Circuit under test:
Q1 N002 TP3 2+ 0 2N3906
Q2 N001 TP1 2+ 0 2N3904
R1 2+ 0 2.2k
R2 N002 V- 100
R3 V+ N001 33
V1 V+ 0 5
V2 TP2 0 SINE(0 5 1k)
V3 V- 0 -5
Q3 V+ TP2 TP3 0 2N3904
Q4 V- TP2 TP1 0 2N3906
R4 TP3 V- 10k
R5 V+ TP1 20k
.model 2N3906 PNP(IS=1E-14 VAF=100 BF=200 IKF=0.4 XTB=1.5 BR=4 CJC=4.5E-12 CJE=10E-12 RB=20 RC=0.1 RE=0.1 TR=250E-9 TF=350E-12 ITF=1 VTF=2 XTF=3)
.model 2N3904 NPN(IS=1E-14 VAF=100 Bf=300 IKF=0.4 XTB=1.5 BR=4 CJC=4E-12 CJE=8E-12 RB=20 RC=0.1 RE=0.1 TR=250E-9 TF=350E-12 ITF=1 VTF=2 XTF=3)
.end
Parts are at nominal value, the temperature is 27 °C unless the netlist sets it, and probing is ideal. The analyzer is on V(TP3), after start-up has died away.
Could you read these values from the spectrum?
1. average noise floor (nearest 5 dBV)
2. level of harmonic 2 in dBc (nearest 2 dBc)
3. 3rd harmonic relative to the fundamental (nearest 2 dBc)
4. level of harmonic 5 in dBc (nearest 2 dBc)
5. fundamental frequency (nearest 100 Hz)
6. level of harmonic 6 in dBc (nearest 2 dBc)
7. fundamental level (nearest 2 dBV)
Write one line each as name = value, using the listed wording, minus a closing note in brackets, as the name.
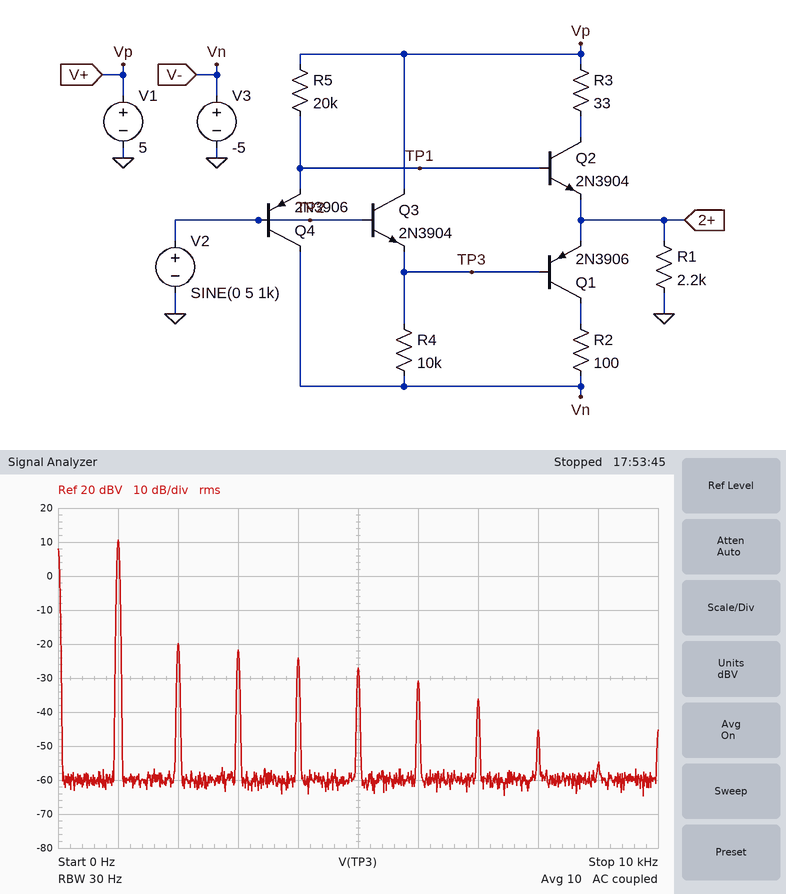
average noise floor = -60 dBV
level of harmonic 2 in dBc = -30 dBc
3rd harmonic relative to the fundamental = -32 dBc
level of harmonic 5 in dBc = -38 dBc
fundamental frequency = 1.0 kHz
level of harmonic 6 in dBc = -42 dBc
fundamental level = 10 dBV
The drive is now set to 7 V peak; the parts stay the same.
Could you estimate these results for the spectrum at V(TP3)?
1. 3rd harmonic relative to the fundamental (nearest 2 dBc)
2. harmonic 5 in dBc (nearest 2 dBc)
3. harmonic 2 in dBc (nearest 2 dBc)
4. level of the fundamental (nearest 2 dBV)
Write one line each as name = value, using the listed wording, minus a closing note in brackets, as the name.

3rd harmonic relative to the fundamental = -18 dBc
harmonic 5 in dBc = -34 dBc
harmonic 2 in dBc = -22 dBc
level of the fundamental = 12 dBV
